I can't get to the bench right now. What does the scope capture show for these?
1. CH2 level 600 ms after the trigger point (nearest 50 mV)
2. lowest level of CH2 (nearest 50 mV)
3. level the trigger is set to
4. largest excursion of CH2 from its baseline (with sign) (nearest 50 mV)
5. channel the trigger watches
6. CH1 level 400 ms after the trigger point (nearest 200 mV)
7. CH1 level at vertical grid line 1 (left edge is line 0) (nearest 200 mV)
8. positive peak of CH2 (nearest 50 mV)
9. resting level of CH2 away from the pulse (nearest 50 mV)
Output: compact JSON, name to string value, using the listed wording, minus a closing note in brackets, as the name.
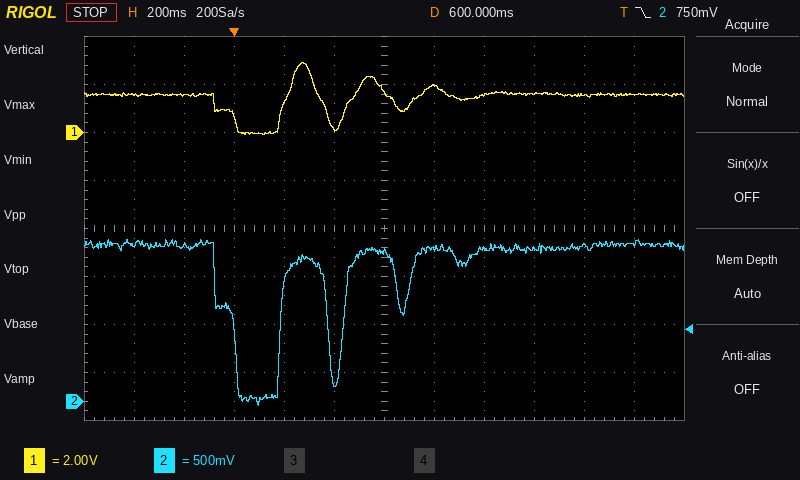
{"CH2 level 600 ms after the trigger point": "1.55 V", "lowest level of CH2": "-50 mV", "level the trigger is set to": "750 mV", "largest excursion of CH2 from its baseline (with sign)": "-1.65 V", "channel the trigger watches": "CH2", "CH1 level 400 ms after the trigger point": "200 mV", "CH1 level at vertical grid line 1 (left edge is line 0)": "1.6 V", "positive peak of CH2": "1.70 V", "resting level of CH2 away from the pulse": "1.60 V"}
